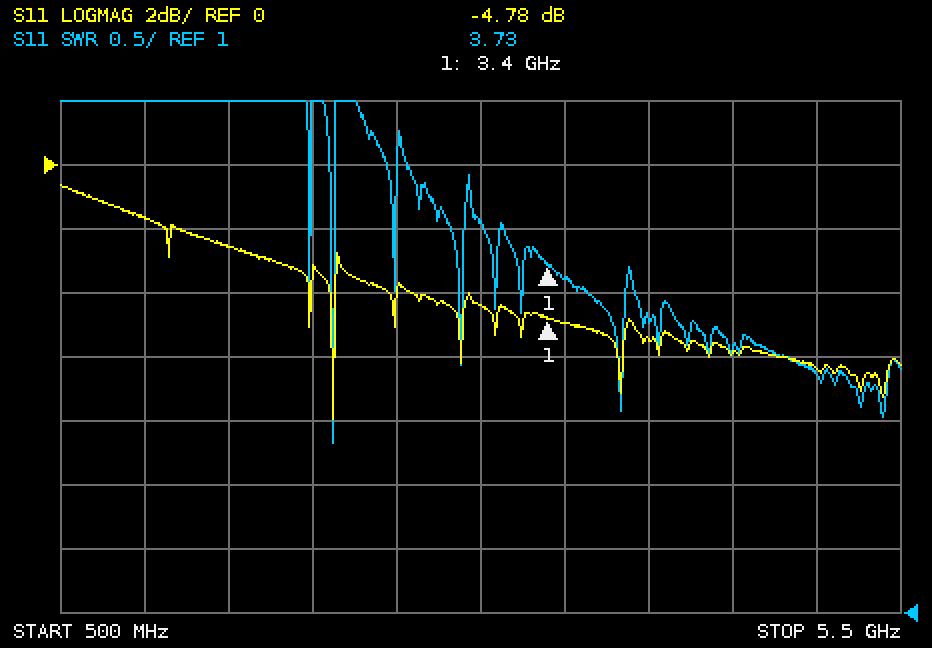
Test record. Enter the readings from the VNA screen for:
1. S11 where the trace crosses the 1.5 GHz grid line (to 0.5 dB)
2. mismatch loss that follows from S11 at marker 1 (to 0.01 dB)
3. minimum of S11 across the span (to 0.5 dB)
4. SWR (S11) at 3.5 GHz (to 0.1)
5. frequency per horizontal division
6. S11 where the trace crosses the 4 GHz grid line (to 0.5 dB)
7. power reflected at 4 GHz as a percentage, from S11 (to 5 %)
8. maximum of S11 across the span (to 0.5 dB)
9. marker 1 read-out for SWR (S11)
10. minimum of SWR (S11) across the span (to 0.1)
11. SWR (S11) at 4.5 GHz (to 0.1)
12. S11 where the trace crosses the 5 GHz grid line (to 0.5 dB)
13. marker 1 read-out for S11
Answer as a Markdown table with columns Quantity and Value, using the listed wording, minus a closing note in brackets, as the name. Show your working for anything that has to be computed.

| Quantity | Value |
|---|---|
| S11 where the trace crosses the 1.5 GHz grid line | -2.5 dB |
| mismatch loss that follows from S11 at marker 1 | −10 log10(1 − 10^(-4.78/10)) ≈ 1.76 dB |
| minimum of S11 across the span | -8.0 dB |
| SWR (S11) at 3.5 GHz | 3.6 |
| frequency per horizontal division | 500 MHz |
| S11 where the trace crosses the 4 GHz grid line | -5.5 dB |
| power reflected at 4 GHz as a percentage, from S11 | 10^(-5.5/10) ≈ 28.2 %, so 30 % to the nearest 5 % |
| maximum of S11 across the span | -0.5 dB |
| marker 1 read-out for SWR | 3.73 |
| minimum of SWR (S11) across the span | 2.3 |
| SWR (S11) at 4.5 GHz | 3.1 |
| S11 where the trace crosses the 5 GHz grid line | -6.5 dB |
| marker 1 read-out for S11 | -4.78 dB |
